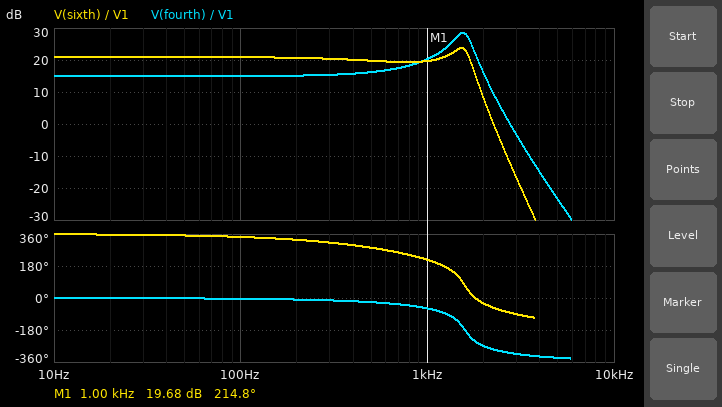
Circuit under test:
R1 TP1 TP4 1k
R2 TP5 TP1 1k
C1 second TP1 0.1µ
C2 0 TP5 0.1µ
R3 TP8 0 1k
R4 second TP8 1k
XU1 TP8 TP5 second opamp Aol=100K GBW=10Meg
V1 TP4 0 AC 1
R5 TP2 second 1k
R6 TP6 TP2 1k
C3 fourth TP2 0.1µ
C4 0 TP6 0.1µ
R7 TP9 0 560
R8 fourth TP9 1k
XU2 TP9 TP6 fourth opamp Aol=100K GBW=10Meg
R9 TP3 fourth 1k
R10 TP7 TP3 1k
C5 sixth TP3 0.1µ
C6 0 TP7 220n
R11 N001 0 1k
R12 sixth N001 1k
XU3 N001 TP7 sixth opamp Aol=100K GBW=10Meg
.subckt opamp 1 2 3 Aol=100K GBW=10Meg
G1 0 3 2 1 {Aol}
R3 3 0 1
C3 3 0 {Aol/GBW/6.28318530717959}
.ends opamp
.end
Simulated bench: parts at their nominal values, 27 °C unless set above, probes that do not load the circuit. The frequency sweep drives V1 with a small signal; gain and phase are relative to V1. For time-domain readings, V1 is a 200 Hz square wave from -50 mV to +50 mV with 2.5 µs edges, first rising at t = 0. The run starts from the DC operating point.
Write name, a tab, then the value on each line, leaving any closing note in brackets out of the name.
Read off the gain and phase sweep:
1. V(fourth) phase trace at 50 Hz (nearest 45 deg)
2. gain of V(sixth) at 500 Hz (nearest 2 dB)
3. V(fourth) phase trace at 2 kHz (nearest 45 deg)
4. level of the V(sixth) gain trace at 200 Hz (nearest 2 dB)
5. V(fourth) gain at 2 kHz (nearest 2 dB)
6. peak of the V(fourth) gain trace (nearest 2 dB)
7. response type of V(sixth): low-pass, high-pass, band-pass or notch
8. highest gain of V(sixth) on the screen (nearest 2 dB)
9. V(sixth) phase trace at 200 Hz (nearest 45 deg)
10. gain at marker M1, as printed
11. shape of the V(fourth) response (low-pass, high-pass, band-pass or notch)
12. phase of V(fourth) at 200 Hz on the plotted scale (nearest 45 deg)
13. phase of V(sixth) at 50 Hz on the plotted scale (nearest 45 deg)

V(fourth) phase trace at 50 Hz	0 deg
gain of V(sixth) at 500 Hz	20 dB
V(fourth) phase trace at 2 kHz	-270 deg
level of the V(sixth) gain trace at 200 Hz	20 dB
V(fourth) gain at 2 kHz	16 dB
peak of the V(fourth) gain trace	28 dB
response type of V(sixth): low-pass, high-pass, band-pass or notch	low-pass
highest gain of V(sixth) on the screen	24 dB
V(sixth) phase trace at 200 Hz	315 deg
gain at marker M1, as printed	19.68 dB
shape of the V(fourth) response	low-pass
phase of V(fourth) at 200 Hz on the plotted scale	0 deg
phase of V(sixth) at 50 Hz on the plotted scale	360 deg
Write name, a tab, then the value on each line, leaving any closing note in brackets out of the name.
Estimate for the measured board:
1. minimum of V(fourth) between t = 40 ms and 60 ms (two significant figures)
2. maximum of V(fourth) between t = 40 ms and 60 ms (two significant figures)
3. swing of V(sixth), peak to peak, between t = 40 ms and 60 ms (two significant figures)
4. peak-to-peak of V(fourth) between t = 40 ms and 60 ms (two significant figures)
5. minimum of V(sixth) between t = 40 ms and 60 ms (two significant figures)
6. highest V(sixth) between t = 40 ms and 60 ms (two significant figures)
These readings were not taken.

minimum of V(fourth) between t = 40 ms and 60 ms	-680 mV
maximum of V(fourth) between t = 40 ms and 60 ms	680 mV
swing of V(sixth), peak to peak, between t = 40 ms and 60 ms	1.3 V
peak-to-peak of V(fourth) between t = 40 ms and 60 ms	1.4 V
minimum of V(sixth) between t = 40 ms and 60 ms	-650 mV
highest V(sixth) between t = 40 ms and 60 ms	650 mV
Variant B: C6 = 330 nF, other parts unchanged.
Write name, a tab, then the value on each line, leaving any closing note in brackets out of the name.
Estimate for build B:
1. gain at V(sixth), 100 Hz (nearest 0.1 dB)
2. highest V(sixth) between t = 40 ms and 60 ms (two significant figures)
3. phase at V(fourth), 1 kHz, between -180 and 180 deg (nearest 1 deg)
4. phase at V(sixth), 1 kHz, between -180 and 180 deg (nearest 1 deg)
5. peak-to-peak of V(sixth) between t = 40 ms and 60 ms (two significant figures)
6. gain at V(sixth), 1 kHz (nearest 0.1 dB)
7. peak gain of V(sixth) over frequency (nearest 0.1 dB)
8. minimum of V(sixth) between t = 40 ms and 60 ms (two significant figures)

gain at V(sixth), 100 Hz	20.6 dB
highest V(sixth) between t = 40 ms and 60 ms	560 mV
phase at V(fourth), 1 kHz, between -180 and 180 deg	-59 deg
phase at V(sixth), 1 kHz, between -180 and 180 deg	-154 deg
peak-to-peak of V(sixth) between t = 40 ms and 60 ms	1.1 V
gain at V(sixth), 1 kHz	15.3 dB
peak gain of V(sixth) over frequency	20.9 dB
minimum of V(sixth) between t = 40 ms and 60 ms	-560 mV
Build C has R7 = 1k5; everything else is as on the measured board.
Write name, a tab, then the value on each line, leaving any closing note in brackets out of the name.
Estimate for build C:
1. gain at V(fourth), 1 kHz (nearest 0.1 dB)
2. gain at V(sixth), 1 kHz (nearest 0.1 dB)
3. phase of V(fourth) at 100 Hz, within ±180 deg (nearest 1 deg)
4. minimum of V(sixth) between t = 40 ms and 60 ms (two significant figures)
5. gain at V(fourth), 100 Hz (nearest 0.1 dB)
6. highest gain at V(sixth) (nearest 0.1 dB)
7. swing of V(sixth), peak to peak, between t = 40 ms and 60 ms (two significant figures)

gain at V(fourth), 1 kHz	11.4 dB
gain at V(sixth), 1 kHz	10.8 dB
phase of V(fourth) at 100 Hz, within ±180 deg	-8 deg
minimum of V(sixth) between t = 40 ms and 60 ms	-330 mV
gain at V(fourth), 100 Hz	10.5 dB
highest gain at V(sixth)	16.5 dB
swing of V(sixth), peak to peak, between t = 40 ms and 60 ms	670 mV
